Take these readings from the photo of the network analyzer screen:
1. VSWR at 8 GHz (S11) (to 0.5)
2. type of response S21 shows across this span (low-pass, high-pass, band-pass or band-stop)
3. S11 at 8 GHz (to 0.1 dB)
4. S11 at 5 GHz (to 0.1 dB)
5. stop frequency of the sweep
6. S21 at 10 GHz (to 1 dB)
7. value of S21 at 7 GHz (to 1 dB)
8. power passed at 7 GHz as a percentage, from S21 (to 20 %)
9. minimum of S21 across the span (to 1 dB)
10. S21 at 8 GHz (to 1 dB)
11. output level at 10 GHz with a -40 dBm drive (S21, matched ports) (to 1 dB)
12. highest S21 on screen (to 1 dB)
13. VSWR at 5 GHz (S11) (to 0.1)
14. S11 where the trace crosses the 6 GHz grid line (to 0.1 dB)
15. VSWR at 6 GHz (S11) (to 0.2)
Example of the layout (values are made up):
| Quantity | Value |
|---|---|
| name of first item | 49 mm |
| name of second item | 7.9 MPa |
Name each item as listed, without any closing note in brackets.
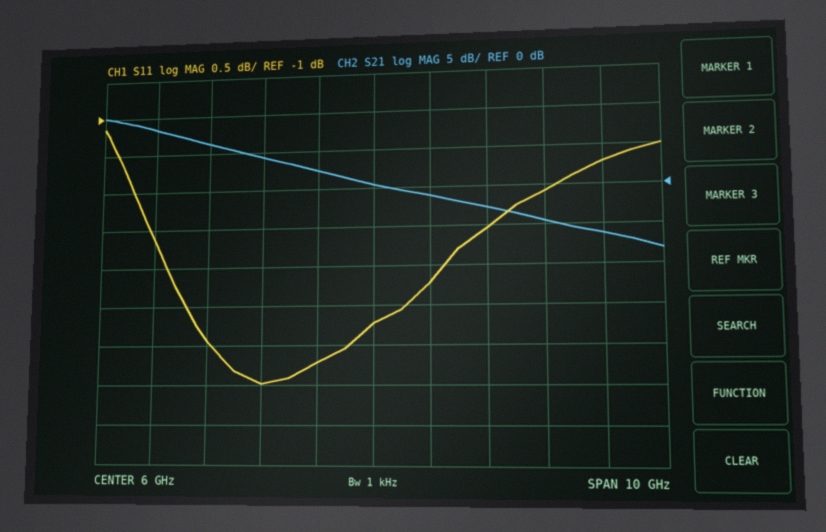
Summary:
| Quantity | Value |
|---|---|
| VSWR at 8 GHz (S11) | 7.0 |
| type of response S21 shows across this span | low-pass |
| S11 at 8 GHz | -2.5 dB |
| S11 at 5 GHz | -4.2 dB |
| stop frequency of the sweep | 11 GHz |
| S21 at 10 GHz | -6 dB |
| value of S21 at 7 GHz | -1 dB |
| power passed at 7 GHz as a percentage, from S21 | 80 % |
| minimum of S21 across the span | -8 dB |
| S21 at 8 GHz | -3 dB |
| output level at 10 GHz with a -40 dBm drive (S21, matched ports) | -46 dBm |
| highest S21 on screen | 10 dB |
| VSWR at 5 GHz (S11) | 4.2 |
| S11 where the trace crosses the 6 GHz grid line | -3.7 dB |
| VSWR at 6 GHz (S11) | 4.8 |
